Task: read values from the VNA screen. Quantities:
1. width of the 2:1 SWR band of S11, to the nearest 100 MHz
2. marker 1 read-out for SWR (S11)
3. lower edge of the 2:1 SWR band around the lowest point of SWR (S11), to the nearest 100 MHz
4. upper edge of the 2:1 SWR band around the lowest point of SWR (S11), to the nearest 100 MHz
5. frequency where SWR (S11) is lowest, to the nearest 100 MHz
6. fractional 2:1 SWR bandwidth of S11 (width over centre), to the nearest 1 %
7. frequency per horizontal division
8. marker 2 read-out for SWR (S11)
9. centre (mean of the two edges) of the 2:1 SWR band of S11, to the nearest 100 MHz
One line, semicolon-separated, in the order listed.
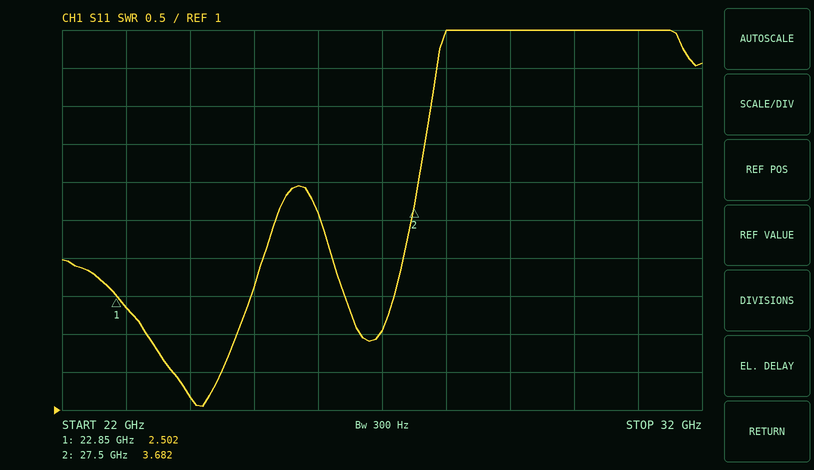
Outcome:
1.4 GHz; 2.502; 23.3 GHz; 24.7 GHz; 24.2 GHz; 6 %; 1 GHz; 3.682; 24.0 GHz
